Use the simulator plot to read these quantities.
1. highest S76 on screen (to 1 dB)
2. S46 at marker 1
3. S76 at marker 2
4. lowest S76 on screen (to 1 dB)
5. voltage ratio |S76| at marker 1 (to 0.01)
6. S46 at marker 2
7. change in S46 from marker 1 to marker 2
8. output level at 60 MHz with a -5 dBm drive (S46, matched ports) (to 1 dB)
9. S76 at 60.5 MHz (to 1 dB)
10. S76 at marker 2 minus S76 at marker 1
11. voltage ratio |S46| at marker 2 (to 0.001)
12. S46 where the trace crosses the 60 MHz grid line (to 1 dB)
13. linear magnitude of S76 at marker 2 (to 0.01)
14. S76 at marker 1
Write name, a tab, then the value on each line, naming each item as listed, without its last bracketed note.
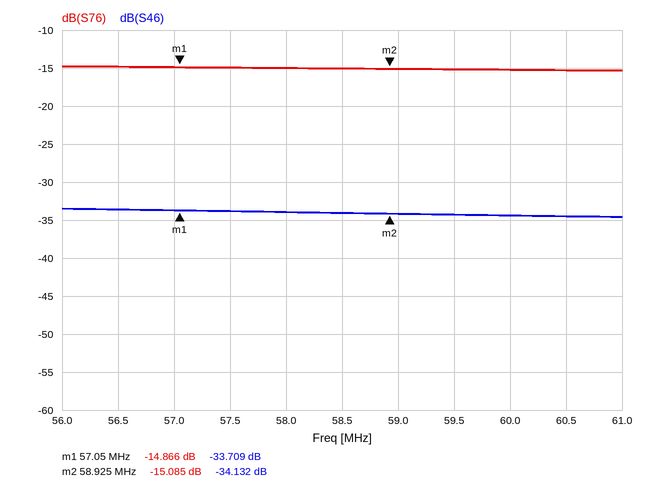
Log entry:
highest S76 on screen	-15 dB
S46 at marker 1	-33.709 dB
S76 at marker 2	-15.085 dB
lowest S76 on screen	-15 dB
voltage ratio |S76| at marker 1	0.18
S46 at marker 2	-34.132 dB
change in S46 from marker 1 to marker 2	-0.423 dB
output level at 60 MHz with a -5 dBm drive (S46, matched ports)	-39 dBm
S76 at 60.5 MHz	-15 dB
S76 at marker 2 minus S76 at marker 1	-0.219 dB
voltage ratio |S46| at marker 2	0.020
S46 where the trace crosses the 60 MHz grid line	-34 dB
linear magnitude of S76 at marker 2	0.18
S76 at marker 1	-14.866 dB
